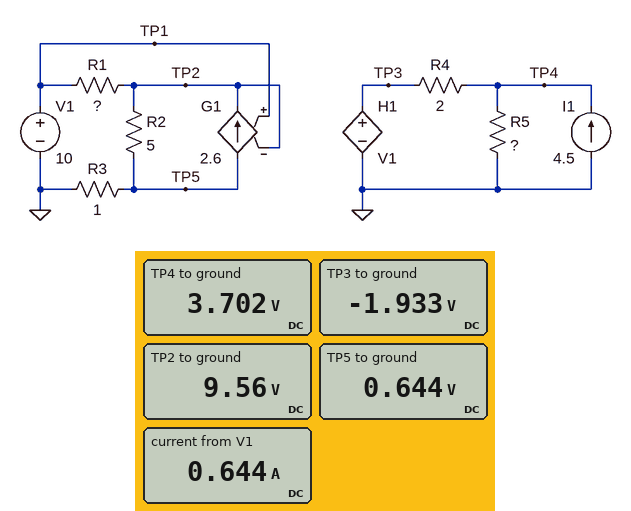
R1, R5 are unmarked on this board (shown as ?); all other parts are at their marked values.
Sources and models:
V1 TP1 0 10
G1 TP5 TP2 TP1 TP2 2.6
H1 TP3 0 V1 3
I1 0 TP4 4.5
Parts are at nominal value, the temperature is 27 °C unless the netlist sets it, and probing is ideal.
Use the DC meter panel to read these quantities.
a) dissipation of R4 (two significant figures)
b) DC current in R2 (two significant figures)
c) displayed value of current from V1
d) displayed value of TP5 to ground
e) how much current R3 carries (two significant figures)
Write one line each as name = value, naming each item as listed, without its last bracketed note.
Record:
dissipation of R4 = 16 W
DC current in R2 = 1.8 A
displayed value of current from V1 = 0.644 A
displayed value of TP5 to ground = 0.644 V
how much current R3 carries = 640 mA
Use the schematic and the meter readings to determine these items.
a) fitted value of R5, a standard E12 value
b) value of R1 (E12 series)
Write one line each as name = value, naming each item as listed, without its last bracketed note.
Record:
fitted value of R5, a standard E12 value = 2.2 Ω
value of R1 = 0.68 Ω
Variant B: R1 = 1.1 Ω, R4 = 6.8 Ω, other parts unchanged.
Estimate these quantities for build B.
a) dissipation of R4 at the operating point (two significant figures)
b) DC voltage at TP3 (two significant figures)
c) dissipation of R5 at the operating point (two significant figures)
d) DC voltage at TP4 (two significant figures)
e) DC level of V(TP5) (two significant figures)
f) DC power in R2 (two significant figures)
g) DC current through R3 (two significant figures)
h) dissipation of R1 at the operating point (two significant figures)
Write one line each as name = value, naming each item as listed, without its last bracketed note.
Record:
dissipation of R4 at the operating point = 11 W
DC voltage at TP3 = -1.4 V
dissipation of R5 at the operating point = 23 W
DC voltage at TP4 = 7.1 V
DC level of V(TP5) = 470 mV
DC power in R2 = 16 W
DC current through R3 = 470 mA
dissipation of R1 at the operating point = 240 mW
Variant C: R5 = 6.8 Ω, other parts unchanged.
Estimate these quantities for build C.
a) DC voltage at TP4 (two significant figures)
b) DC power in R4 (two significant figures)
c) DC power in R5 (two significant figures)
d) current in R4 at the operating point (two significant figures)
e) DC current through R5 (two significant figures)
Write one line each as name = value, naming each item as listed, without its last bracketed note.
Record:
DC voltage at TP4 = 5.5 V
DC power in R4 = 27 W
DC power in R5 = 4.4 W
current in R4 at the operating point = 3.7 A
DC current through R5 = 800 mA
